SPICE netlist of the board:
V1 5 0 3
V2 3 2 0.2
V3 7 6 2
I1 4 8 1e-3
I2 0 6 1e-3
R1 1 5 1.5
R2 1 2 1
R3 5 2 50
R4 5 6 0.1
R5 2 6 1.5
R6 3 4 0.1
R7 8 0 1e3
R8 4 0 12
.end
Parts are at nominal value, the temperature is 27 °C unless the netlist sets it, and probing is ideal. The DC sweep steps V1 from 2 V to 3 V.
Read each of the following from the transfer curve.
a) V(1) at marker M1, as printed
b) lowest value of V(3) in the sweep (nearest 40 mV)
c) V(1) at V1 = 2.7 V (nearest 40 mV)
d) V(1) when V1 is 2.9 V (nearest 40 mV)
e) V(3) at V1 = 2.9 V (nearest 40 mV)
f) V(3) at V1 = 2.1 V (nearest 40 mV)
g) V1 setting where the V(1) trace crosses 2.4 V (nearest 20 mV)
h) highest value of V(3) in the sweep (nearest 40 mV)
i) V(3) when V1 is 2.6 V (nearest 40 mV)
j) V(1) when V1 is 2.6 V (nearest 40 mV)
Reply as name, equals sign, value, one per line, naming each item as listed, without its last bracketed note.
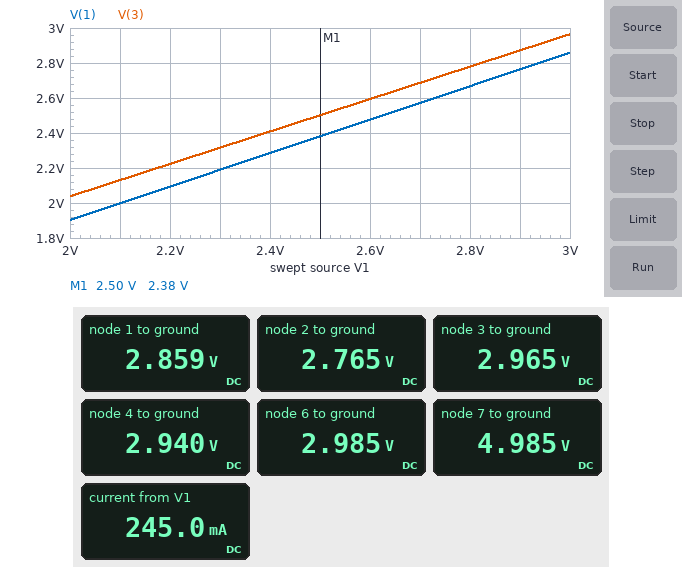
V(1) at marker M1, as printed = 2.38 V
lowest value of V(3) in the sweep = 2.04 V
V(1) at V1 = 2.7 V = 2.56 V
V(1) when V1 is 2.9 V = 2.76 V
V(3) at V1 = 2.9 V = 2.88 V
V(3) at V1 = 2.1 V = 2.12 V
V1 setting where the V(1) trace crosses 2.4 V = 2.52 V
highest value of V(3) in the sweep = 2.96 V
V(3) when V1 is 2.6 V = 2.60 V
V(1) when V1 is 2.6 V = 2.48 V
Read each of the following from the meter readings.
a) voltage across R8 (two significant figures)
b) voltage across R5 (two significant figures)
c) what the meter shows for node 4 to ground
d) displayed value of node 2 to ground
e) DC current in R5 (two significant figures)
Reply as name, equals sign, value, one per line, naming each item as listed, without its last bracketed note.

voltage across R8 = 2.9 V
voltage across R5 = 220 mV
what the meter shows for node 4 to ground = 2.940 V
displayed value of node 2 to ground = 2.765 V
DC current in R5 = 150 mA
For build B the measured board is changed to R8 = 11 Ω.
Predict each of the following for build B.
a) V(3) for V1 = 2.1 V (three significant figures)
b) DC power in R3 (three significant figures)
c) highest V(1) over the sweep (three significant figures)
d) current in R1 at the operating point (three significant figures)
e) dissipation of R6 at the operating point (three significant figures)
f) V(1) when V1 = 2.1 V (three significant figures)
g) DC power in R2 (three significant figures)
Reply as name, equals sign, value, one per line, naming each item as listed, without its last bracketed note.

V(3) for V1 = 2.1 V = 2.12 V
DC power in R3 = 1.30 mW
highest V(1) over the sweep = 2.85 V
current in R1 at the operating point = 102 mA
dissipation of R6 at the operating point = 7.09 mW
V(1) when V1 = 2.1 V = 1.99 V
DC power in R2 = 10.4 mW
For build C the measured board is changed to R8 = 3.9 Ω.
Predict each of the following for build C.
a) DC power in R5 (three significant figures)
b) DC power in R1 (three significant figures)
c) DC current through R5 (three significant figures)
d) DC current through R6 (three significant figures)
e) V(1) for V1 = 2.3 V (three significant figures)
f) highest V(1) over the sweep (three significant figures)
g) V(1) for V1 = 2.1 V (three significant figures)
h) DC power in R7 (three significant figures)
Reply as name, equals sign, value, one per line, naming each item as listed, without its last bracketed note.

DC power in R5 = 224 mW
DC power in R1 = 91.8 mW
DC current through R5 = 387 mA
DC current through R6 = 646 mA
V(1) for V1 = 2.3 V = 2.01 V
highest V(1) over the sweep = 2.63 V
V(1) for V1 = 2.1 V = 1.83 V
DC power in R7 = 1.00 mW
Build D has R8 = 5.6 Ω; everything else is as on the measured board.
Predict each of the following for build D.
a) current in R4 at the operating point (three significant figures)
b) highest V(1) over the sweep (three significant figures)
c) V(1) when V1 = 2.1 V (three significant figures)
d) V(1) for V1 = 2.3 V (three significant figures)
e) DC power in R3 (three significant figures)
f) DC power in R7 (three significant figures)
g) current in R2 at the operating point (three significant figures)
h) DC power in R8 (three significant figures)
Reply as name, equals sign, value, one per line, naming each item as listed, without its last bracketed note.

current in R4 at the operating point = 287 mA
highest V(1) over the sweep = 2.72 V
V(1) when V1 = 2.1 V = 1.90 V
V(1) for V1 = 2.3 V = 2.08 V
DC power in R3 = 4.25 mW
DC power in R7 = 1.00 mW
current in R2 at the operating point = 184 mA
DC power in R8 = 1.29 W
